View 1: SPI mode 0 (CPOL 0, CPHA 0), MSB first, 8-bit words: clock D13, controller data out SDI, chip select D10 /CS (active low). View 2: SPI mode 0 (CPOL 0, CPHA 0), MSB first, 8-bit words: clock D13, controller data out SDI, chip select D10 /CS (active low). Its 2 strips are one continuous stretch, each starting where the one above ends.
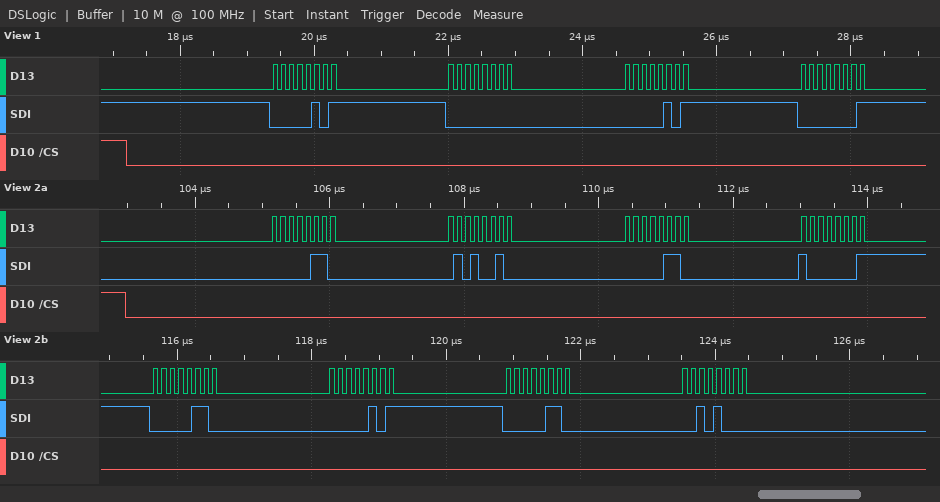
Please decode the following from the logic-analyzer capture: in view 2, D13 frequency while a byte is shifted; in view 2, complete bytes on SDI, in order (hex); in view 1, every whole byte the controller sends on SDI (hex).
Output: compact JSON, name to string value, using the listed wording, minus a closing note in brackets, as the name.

{"in view 2, D13 frequency while a byte is shifted": "8 MHz", "in view 2, complete bytes on SDI, in order": "06 52 06 81 06 05 06 28", "in view 1, every whole byte the controller sends on SDI": "0x05 0x00 0x05 0x01"}
